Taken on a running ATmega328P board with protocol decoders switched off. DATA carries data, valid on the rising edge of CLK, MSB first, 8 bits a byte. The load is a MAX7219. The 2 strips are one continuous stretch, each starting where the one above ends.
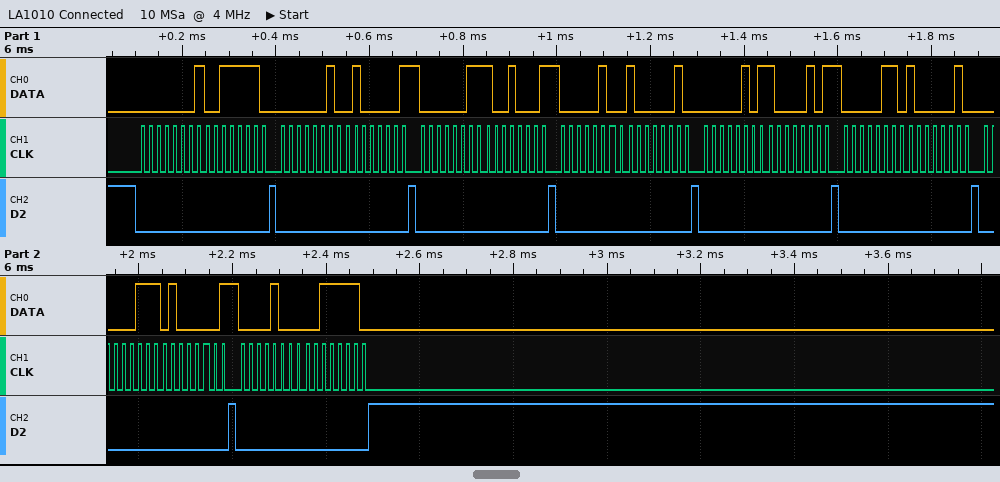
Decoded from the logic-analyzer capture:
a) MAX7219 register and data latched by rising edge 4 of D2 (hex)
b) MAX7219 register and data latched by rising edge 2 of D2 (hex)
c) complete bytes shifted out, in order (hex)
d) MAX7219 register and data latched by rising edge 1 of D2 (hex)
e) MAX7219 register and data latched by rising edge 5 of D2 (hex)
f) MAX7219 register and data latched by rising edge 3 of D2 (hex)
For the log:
register 0x4, data 0x82
register 0x2, data 0x41
01 3E 02 41 03 91 04 82 05 85 06 82 07 41 08 3E
register 0x1, data 0x3E
register 0x5, data 0x85
register 0x3, data 0x91
